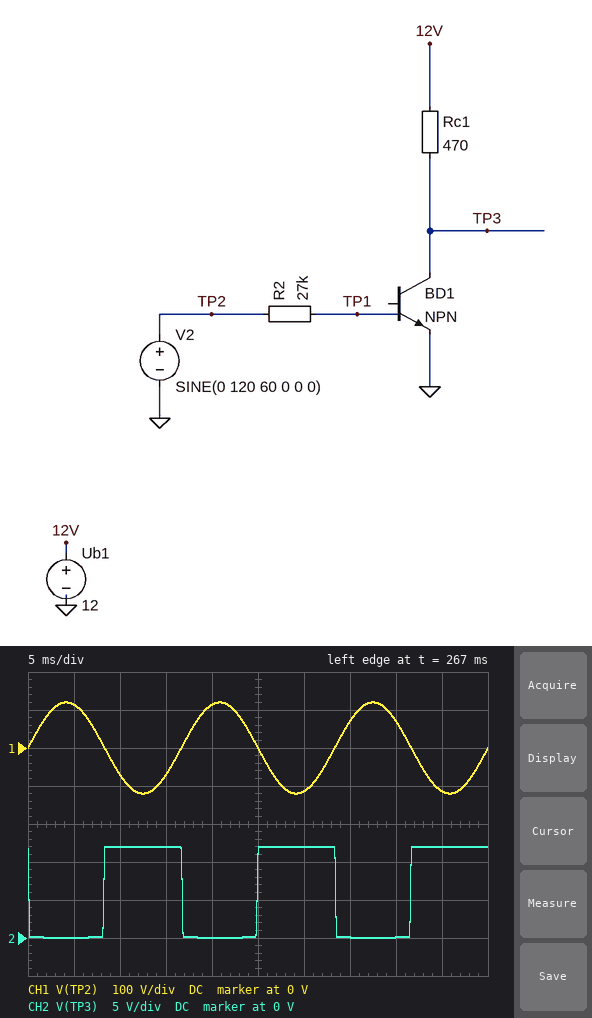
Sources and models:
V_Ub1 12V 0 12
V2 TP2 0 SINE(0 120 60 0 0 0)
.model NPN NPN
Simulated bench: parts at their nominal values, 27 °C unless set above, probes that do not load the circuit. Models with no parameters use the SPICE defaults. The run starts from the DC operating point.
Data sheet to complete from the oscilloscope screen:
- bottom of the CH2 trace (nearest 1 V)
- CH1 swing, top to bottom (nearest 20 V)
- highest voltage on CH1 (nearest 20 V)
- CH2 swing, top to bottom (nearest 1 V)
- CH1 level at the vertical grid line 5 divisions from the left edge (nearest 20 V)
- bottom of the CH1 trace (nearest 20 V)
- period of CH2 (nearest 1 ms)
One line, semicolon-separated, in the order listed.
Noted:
0 V; 240 V; 120 V; 12 V; 0 V; -120 V; 17 ms
